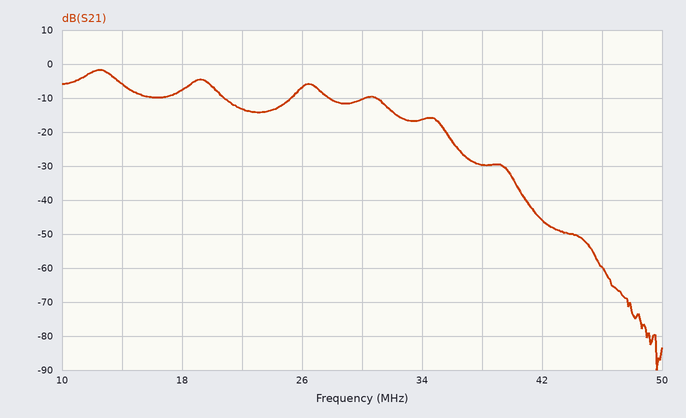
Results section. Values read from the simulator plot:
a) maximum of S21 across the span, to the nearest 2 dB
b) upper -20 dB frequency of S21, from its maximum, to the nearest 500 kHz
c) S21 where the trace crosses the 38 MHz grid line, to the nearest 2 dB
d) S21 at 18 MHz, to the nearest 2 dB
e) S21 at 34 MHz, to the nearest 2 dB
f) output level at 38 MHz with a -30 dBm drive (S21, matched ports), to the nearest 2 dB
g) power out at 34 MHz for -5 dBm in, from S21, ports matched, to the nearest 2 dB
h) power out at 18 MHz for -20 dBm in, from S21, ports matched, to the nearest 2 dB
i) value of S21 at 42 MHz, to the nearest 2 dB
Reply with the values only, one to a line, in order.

-2 dB
36.0 MHz
-30 dB
-8 dB
-16 dB
-60 dBm
-22 dBm
-28 dBm
-46 dB
